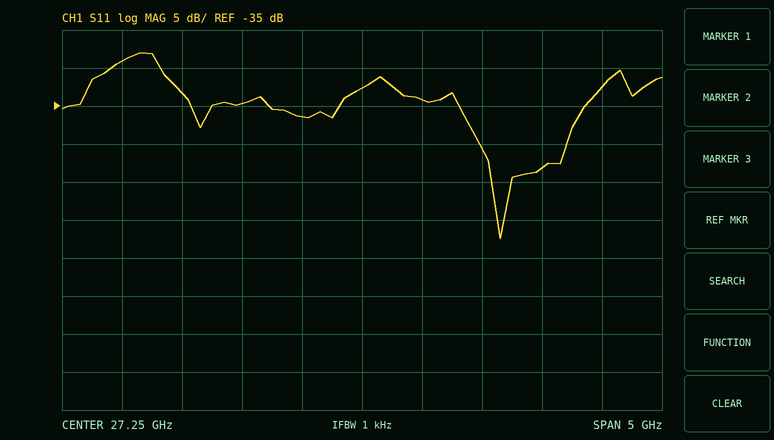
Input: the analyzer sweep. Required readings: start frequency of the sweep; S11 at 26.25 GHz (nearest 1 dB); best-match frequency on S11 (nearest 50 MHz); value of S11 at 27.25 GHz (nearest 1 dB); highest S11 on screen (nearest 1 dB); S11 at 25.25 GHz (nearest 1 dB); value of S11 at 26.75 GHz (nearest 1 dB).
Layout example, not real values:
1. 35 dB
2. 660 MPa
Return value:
1. 24.75 GHz
2. -35 dB
3. 28.40 GHz
4. -33 dB
5. -28 dB
6. -29 dB
7. -36 dB
